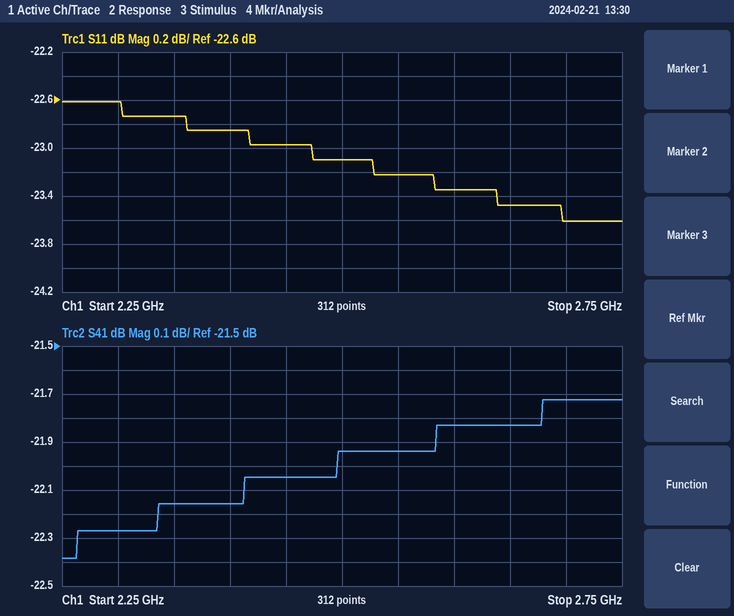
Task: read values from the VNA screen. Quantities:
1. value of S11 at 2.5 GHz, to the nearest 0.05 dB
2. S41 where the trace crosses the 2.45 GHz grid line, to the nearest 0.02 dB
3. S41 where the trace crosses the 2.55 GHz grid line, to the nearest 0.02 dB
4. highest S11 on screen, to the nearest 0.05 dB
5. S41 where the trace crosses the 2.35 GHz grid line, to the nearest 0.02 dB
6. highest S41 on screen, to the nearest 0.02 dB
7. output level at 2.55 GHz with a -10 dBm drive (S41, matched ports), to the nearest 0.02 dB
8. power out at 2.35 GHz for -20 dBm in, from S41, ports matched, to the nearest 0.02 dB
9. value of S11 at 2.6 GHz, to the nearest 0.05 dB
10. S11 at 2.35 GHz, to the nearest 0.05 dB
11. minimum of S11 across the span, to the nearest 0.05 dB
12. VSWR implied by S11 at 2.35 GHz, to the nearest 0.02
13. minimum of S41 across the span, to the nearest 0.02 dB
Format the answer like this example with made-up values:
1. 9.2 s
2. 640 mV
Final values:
1. -23.10 dB
2. -22.04 dB
3. -21.94 dB
4. -22.60 dB
5. -22.16 dB
6. -21.72 dB
7. -31.94 dBm
8. -42.16 dBm
9. -23.35 dB
10. -22.75 dB
11. -23.60 dB
12. 1.16
13. -22.38 dB
